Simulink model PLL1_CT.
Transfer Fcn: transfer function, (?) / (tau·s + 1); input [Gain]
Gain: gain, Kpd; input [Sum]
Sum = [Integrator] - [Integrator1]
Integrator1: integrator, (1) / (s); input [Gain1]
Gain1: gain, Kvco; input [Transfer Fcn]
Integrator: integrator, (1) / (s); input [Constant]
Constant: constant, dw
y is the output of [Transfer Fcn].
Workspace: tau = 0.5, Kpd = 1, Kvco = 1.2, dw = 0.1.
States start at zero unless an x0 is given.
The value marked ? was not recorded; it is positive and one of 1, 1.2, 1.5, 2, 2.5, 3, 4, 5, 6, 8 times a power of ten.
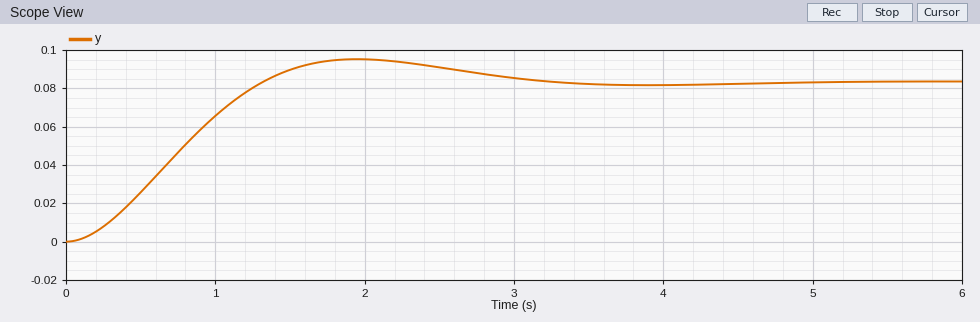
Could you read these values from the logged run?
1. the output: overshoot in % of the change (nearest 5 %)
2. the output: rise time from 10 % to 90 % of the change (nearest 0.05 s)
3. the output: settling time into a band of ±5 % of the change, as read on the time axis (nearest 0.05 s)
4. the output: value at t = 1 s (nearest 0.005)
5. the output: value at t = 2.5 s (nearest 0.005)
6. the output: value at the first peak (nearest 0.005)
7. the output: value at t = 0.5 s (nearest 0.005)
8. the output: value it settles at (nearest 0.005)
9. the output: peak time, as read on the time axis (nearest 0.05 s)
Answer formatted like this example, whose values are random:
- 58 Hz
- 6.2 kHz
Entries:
- 15 %
- 0.90 s
- 2.80 s
- 0.065
- 0.090
- 0.095
- 0.025
- 0.085
- 1.95 s
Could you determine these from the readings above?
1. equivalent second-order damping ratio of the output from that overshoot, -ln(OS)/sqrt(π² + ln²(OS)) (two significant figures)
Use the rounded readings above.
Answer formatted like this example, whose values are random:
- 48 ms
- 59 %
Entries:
- 0.52
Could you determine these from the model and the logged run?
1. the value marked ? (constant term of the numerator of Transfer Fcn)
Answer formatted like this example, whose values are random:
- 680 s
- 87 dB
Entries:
- 1.5
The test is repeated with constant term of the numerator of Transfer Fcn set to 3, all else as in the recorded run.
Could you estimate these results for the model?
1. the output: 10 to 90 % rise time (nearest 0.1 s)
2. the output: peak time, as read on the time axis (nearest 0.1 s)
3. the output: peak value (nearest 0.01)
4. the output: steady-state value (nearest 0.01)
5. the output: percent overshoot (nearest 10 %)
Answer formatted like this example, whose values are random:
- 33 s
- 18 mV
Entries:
- 0.5 s
- 1.3 s
- 0.11
- 0.08
- 30 %
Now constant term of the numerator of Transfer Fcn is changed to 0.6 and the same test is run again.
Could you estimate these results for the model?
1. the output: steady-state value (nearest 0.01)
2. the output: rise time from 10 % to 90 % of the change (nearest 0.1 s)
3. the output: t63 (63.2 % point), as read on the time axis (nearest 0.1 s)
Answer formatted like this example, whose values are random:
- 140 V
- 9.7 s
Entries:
- 0.08
- 2.2 s
- 1.6 s
